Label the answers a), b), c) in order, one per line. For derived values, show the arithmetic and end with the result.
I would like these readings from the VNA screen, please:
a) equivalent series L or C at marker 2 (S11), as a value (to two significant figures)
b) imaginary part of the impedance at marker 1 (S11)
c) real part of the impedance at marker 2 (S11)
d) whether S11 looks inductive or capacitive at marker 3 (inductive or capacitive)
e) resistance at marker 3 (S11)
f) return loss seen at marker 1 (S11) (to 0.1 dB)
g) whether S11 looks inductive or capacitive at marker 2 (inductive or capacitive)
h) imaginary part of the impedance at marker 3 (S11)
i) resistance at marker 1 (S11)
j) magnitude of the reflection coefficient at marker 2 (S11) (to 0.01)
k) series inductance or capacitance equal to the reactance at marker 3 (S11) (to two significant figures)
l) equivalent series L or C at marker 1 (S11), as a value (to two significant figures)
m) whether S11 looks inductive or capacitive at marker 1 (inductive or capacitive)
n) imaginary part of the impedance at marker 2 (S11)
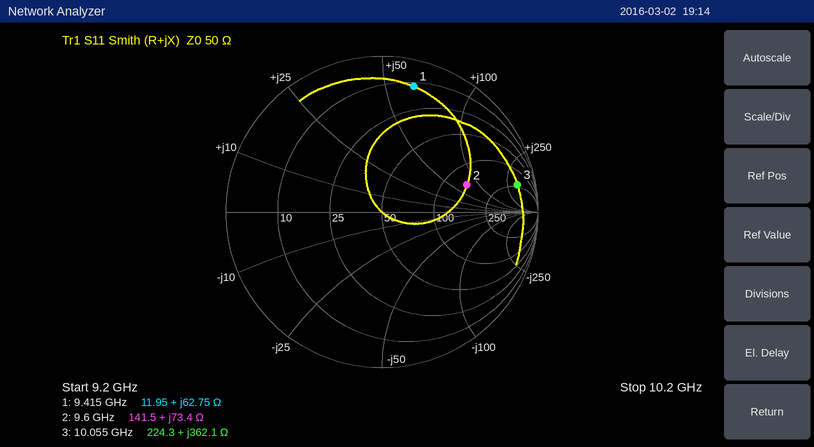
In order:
a) L = 73.4 Ω/(2π × 9.6 GHz) ≈ 1.2 nH
b) +62.75 Ω
c) 141.5 Ω
d) inductive
e) 224.3 Ω
f) 1.6 dB
g) inductive
h) +362.1 Ω
i) 11.95 Ω
j) 0.57
k) L = 362.1 Ω/(2π × 10.055 GHz) ≈ 5.7 nH
l) L = 62.75 Ω/(2π × 9.415 GHz) ≈ 1.1 nH
m) inductive
n) +73.4 Ω
